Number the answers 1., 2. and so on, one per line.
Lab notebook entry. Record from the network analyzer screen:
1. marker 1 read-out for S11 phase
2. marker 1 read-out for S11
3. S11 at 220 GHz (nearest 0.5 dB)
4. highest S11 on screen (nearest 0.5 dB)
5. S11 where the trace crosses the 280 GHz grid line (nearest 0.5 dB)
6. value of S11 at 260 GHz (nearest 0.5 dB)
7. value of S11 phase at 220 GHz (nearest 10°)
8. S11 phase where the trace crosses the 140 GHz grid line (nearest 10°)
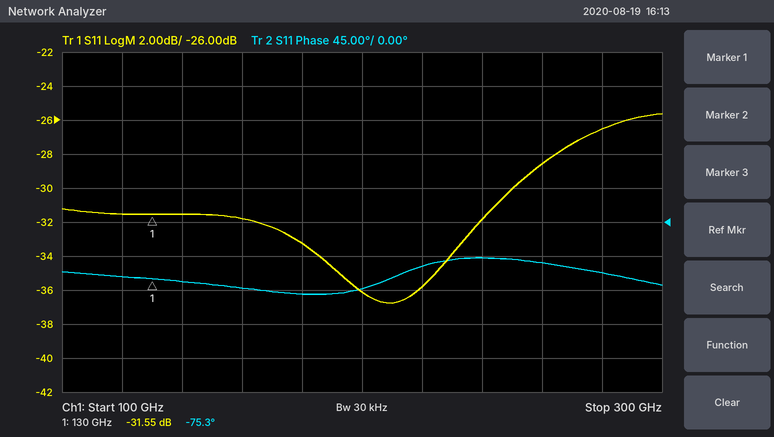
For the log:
1. -75.3°
2. -31.55 dB
3. -36.0 dB
4. -25.5 dB
5. -26.5 dB
6. -28.5 dB
7. -60°
8. -80°
